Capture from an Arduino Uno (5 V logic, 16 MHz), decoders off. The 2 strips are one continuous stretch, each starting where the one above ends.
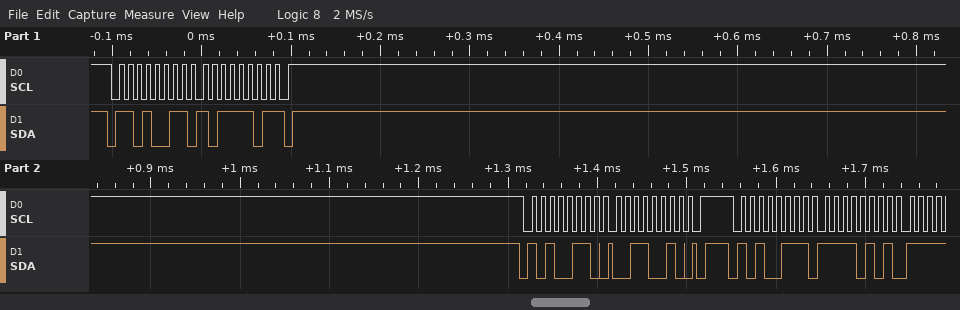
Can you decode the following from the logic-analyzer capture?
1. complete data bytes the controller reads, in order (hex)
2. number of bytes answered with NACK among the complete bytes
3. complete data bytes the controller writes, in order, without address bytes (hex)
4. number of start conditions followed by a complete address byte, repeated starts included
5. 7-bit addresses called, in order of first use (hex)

BD F5
1
32
3
0x69 0x53
